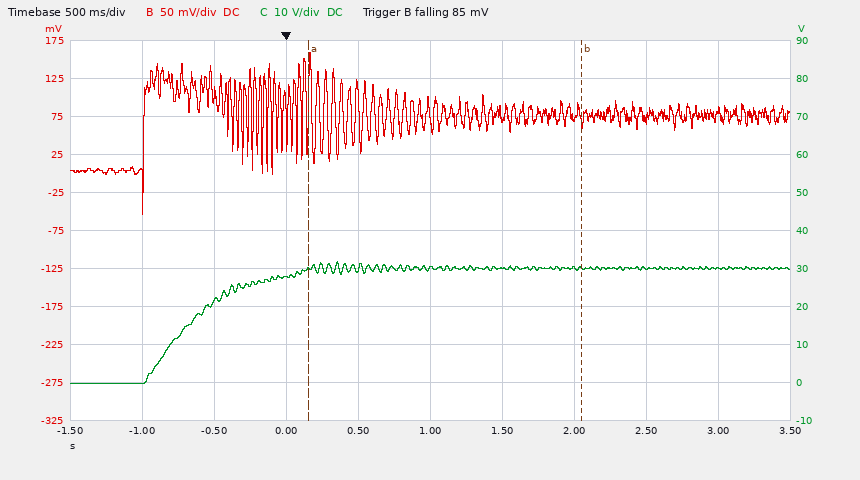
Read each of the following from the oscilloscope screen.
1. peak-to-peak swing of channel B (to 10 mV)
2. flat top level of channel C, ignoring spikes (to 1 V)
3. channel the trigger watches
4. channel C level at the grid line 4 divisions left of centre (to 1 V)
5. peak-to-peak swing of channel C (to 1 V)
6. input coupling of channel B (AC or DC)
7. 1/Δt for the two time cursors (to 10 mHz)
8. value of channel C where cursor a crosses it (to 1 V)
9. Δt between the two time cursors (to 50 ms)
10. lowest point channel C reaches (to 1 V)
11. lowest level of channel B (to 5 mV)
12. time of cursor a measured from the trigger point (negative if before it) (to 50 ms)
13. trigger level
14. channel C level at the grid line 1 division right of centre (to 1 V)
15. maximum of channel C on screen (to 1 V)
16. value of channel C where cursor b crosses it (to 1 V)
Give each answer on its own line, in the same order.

210 mV
30 V
channel B
0 V
32 V
DC
530 mHz
30 V
1.90 s
0 V
-55 mV
+150 ms
85 mV
30 V
32 V
30 V
